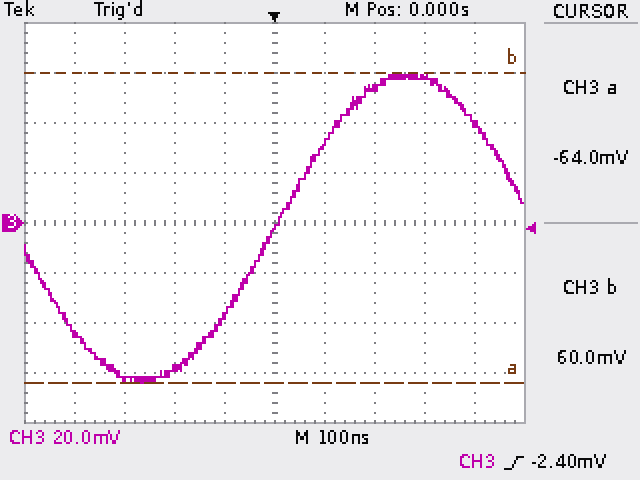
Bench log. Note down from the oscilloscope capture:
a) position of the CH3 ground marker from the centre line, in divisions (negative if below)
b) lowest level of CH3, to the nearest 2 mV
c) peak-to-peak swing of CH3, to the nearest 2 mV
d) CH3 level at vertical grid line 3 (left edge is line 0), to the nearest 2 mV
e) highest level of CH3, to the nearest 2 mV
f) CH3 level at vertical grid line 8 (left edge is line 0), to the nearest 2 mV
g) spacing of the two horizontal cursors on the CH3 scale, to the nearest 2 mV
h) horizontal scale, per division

0.0 div
-64 mV
124 mV
-58 mV
60 mV
58 mV
124 mV
100 ns
